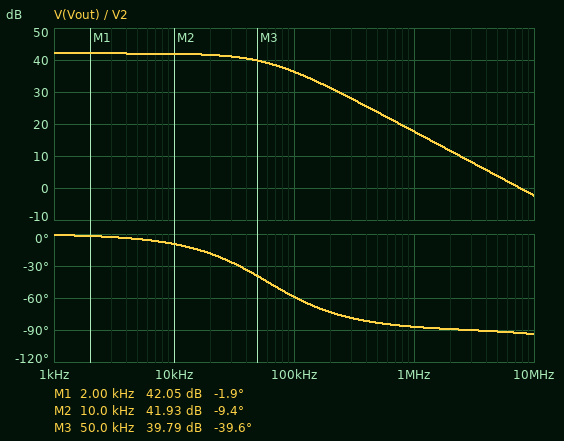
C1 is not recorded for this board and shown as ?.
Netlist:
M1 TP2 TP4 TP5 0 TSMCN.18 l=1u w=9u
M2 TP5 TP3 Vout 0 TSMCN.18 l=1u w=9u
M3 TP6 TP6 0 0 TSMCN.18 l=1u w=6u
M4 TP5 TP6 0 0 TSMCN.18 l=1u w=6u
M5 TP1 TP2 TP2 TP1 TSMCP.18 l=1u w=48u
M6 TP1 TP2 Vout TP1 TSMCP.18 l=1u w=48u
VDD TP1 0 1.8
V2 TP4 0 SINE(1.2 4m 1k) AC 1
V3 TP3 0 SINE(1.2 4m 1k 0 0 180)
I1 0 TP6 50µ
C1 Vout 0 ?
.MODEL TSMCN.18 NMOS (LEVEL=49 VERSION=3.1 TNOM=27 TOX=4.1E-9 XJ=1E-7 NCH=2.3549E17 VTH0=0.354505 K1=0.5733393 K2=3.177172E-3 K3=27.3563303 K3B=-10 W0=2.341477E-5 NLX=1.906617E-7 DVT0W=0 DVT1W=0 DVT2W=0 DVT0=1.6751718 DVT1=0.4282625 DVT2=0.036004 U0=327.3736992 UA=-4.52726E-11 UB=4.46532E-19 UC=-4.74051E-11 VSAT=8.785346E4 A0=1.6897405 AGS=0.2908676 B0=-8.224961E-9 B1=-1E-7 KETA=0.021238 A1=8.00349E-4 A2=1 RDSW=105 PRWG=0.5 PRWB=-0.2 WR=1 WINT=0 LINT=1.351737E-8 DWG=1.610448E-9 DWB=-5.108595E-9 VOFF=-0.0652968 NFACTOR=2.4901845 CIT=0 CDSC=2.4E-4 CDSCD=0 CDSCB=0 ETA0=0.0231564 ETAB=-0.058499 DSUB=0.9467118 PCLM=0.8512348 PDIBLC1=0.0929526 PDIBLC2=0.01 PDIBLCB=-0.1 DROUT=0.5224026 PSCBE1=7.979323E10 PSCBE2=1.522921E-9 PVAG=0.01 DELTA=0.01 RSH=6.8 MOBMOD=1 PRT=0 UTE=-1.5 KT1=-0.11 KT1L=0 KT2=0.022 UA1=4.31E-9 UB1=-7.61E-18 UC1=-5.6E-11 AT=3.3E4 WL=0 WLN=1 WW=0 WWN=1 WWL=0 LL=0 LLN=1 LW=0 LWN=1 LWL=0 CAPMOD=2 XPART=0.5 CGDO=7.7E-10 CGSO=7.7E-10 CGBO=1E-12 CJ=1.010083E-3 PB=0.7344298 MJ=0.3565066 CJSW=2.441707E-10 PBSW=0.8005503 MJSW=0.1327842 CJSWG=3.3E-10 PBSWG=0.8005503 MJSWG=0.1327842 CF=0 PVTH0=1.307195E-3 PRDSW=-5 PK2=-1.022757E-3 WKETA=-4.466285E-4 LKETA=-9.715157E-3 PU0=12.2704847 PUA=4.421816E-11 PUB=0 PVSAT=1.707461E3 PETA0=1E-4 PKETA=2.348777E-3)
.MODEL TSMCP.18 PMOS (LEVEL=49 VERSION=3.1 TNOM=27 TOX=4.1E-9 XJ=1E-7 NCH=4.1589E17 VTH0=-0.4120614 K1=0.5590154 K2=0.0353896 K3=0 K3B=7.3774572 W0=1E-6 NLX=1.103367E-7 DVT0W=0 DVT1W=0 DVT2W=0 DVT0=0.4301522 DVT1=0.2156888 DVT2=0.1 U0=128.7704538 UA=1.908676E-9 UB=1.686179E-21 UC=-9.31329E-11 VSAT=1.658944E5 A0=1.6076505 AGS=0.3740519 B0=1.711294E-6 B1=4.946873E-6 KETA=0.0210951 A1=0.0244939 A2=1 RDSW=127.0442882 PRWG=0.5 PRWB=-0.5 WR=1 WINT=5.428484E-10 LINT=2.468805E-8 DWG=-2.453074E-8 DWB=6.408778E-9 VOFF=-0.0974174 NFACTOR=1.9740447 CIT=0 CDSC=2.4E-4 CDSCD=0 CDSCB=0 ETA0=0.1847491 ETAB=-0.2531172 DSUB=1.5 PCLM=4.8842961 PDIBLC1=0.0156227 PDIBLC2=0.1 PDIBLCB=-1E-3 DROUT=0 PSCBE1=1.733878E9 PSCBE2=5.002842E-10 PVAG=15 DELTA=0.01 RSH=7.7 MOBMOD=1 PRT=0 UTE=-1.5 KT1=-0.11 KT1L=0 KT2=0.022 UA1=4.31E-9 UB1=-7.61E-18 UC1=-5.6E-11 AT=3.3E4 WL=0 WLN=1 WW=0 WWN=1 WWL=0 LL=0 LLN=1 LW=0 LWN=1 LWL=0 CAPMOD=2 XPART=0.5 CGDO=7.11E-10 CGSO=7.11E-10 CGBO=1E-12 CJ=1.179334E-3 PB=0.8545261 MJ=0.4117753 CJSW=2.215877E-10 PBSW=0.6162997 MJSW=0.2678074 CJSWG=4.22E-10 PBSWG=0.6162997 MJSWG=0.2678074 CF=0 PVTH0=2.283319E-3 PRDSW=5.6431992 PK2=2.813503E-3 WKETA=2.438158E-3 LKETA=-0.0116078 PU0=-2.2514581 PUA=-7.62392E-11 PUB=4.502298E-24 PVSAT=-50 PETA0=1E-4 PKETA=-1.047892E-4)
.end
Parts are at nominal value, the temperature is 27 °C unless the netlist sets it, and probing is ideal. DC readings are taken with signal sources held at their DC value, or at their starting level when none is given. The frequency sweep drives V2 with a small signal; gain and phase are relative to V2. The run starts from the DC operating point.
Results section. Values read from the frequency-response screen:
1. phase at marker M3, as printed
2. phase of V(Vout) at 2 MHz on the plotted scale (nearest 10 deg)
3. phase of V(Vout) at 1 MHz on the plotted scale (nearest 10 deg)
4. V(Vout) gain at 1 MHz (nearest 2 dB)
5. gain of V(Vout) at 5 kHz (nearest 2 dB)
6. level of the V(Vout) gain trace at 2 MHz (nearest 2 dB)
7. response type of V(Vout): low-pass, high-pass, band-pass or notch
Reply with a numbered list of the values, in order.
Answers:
1. -39.6 deg
2. -90 deg
3. -90 deg
4. 18 dB
5. 42 dB
6. 12 dB
7. low-pass
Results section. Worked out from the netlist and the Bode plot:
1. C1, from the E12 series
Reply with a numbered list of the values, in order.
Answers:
1. 6.8 pF
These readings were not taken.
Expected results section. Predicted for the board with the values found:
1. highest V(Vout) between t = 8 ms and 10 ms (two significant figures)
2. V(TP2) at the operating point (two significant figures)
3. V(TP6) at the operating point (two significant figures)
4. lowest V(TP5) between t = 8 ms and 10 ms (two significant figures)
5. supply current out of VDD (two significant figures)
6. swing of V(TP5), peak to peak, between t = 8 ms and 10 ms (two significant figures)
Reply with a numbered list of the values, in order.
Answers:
1. 1.7 V
2. 1.2 V
3. 690 mV
4. 490 mV
5. 49 µA
6. 3.5 mV
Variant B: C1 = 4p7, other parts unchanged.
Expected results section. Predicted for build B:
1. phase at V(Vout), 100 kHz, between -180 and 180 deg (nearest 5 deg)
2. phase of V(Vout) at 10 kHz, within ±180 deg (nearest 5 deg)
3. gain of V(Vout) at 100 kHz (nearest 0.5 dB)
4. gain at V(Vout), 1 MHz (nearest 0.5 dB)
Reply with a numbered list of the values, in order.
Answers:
1. -50 deg
2. -5 deg
3. 38.5 dB
4. 21.0 dB
